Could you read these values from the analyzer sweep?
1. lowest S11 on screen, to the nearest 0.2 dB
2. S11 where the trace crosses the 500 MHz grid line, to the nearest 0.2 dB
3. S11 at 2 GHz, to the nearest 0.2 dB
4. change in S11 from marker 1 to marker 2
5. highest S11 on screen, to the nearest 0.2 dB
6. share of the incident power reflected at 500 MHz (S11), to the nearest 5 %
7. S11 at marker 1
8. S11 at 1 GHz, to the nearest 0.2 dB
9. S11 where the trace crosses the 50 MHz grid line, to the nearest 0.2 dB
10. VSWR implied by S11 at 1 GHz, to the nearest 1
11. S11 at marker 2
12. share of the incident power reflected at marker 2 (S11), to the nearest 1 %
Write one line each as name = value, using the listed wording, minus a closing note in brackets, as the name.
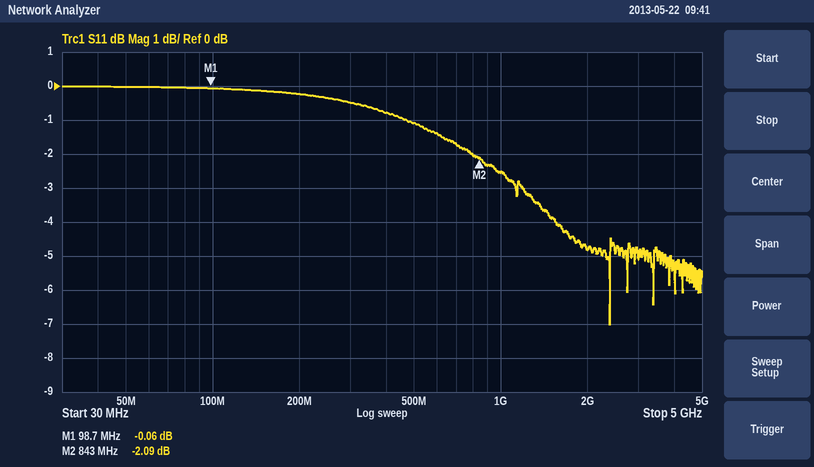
lowest S11 on screen, to the nearest 0.2 dB = -7.0 dB
S11 where the trace crosses the 500 MHz grid line, to the nearest 0.2 dB = -1.0 dB
S11 at 2 GHz, to the nearest 0.2 dB = -4.8 dB
change in S11 from marker 1 to marker 2 = -2.03 dB
highest S11 on screen, to the nearest 0.2 dB = 0.0 dB
share of the incident power reflected at 500 MHz (S11), to the nearest 5 % = 80 %
S11 at marker 1 = -0.06 dB
S11 at 1 GHz, to the nearest 0.2 dB = -2.6 dB
S11 where the trace crosses the 50 MHz grid line, to the nearest 0.2 dB = 0.0 dB
VSWR implied by S11 at 1 GHz, to the nearest 1 = 7
S11 at marker 2 = -2.09 dB
share of the incident power reflected at marker 2 (S11), to the nearest 1 % = 62 %
